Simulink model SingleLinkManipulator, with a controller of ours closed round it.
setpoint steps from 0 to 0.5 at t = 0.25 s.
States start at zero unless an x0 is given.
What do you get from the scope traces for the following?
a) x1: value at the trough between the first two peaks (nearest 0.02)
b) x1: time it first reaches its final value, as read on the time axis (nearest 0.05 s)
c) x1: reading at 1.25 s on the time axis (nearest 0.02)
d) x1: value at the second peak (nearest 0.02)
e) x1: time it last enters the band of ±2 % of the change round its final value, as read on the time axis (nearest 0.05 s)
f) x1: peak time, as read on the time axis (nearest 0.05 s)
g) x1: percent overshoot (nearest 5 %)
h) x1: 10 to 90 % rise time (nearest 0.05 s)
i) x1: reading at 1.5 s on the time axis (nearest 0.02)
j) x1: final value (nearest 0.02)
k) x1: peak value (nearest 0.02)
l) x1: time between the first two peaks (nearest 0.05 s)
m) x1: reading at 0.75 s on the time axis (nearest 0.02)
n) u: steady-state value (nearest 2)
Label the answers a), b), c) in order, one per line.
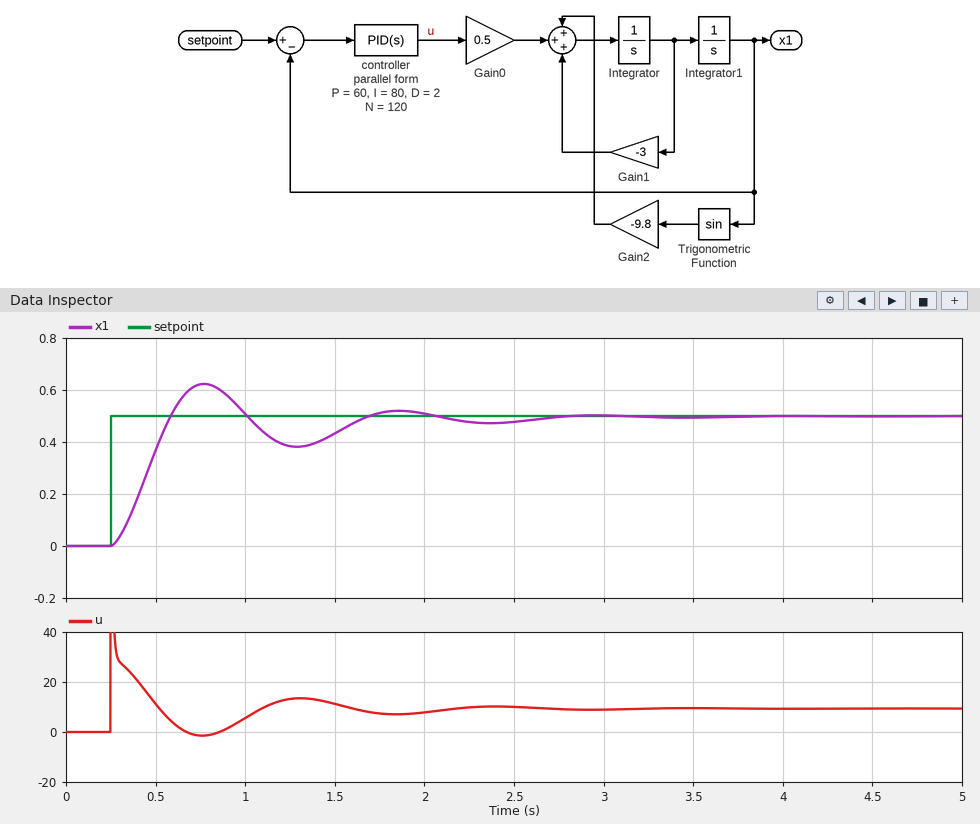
a) 0.38
b) 0.60 s
c) 0.38
d) 0.52
e) 2.65 s
f) 0.75 s
g) 25 %
h) 0.25 s
i) 0.44
j) 0.50
k) 0.62
l) 1.10 s
m) 0.62
n) 10
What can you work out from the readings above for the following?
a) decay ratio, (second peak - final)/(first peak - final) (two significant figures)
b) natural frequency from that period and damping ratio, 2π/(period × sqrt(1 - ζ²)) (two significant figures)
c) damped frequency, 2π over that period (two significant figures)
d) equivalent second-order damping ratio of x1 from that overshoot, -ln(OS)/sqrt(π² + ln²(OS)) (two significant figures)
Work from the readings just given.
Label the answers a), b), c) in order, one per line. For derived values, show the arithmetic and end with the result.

a) (0.52 - 0.5) / (0.62 - 0.5) = 0.17
b) 2π / (1.1 × sqrt(1 - 0.4²)) = 6.2 rad/s
c) 2π / 1.1 = 5.7 rad/s
d) ln(0.25) = -1.386; 1.386 / sqrt(9.870 + 1.922) = 0.40
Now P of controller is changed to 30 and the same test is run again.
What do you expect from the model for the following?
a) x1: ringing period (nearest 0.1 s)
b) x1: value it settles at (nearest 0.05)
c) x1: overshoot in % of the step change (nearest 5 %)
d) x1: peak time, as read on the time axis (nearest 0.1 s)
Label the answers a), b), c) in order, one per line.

a) 1.4 s
b) 0.50
c) 20 %
d) 1.0 s
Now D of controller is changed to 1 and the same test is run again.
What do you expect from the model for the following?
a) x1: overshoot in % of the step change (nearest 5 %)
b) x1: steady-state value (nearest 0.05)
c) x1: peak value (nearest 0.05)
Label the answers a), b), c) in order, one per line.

a) 30 %
b) 0.50
c) 0.65
